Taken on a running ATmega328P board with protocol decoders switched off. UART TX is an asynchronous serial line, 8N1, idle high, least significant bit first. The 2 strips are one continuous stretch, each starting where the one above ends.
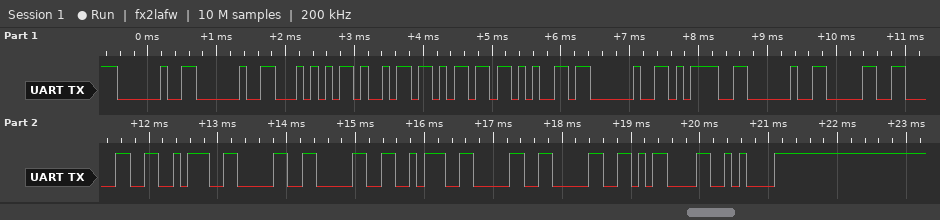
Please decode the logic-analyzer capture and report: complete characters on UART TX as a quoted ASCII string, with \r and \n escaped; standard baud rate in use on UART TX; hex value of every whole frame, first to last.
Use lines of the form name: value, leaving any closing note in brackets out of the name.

complete characters on UART TX as a quoted ASCII string, with \r and \n escaped: "  Time = 00:00:00\r\n"
standard baud rate in use on UART TX: 9600 baud
hex value of every whole frame, first to last: 20 20 54 69 6D 65 20 3D 20 30 30 3A 30 30 3A 30 30 0D 0A
